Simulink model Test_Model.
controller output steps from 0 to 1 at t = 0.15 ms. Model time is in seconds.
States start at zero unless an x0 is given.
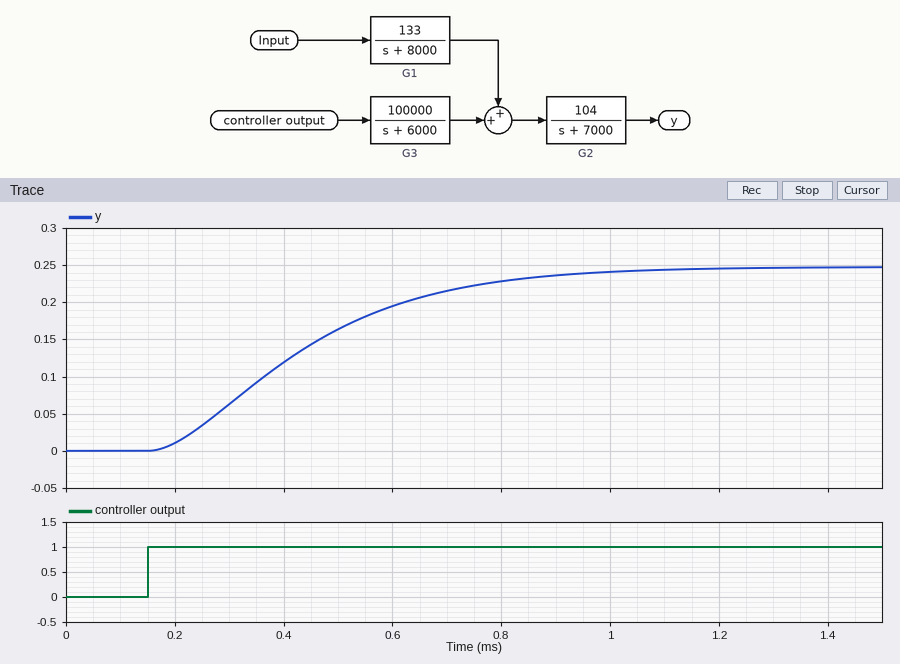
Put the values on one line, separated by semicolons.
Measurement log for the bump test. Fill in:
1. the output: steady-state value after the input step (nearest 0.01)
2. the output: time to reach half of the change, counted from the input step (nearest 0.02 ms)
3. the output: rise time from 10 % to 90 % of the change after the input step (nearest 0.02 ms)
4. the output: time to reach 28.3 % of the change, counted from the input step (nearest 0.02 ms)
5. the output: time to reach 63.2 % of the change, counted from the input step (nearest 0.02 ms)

0.25; 0.26 ms; 0.52 ms; 0.16 ms; 0.34 ms
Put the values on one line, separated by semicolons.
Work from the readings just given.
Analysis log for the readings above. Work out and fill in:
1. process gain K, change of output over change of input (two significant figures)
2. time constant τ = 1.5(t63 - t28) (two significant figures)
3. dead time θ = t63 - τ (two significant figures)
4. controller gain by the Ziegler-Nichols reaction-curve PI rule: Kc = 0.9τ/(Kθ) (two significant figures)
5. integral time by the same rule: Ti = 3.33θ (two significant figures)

0.25; 0.27 ms; 0.070 ms; 14; 0.23 ms
